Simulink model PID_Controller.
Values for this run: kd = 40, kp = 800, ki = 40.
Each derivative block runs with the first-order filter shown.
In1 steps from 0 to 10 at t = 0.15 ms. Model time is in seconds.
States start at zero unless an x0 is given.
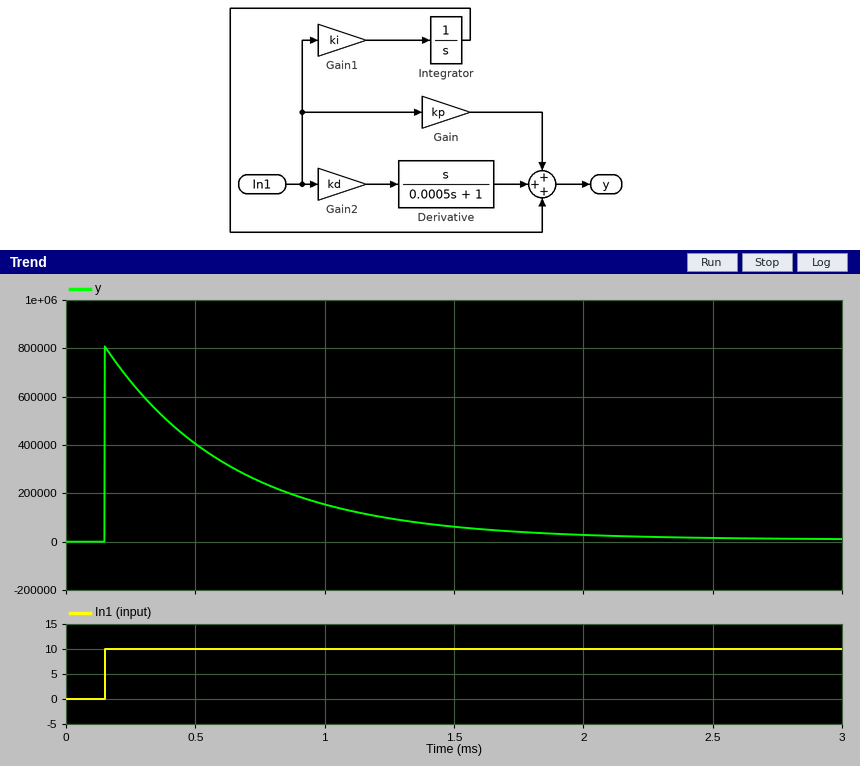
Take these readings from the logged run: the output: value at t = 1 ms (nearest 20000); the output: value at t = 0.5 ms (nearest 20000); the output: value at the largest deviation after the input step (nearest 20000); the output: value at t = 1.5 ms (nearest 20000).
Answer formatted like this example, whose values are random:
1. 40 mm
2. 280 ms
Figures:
1. 160000
2. 400000
3. 800000
4. 60000
